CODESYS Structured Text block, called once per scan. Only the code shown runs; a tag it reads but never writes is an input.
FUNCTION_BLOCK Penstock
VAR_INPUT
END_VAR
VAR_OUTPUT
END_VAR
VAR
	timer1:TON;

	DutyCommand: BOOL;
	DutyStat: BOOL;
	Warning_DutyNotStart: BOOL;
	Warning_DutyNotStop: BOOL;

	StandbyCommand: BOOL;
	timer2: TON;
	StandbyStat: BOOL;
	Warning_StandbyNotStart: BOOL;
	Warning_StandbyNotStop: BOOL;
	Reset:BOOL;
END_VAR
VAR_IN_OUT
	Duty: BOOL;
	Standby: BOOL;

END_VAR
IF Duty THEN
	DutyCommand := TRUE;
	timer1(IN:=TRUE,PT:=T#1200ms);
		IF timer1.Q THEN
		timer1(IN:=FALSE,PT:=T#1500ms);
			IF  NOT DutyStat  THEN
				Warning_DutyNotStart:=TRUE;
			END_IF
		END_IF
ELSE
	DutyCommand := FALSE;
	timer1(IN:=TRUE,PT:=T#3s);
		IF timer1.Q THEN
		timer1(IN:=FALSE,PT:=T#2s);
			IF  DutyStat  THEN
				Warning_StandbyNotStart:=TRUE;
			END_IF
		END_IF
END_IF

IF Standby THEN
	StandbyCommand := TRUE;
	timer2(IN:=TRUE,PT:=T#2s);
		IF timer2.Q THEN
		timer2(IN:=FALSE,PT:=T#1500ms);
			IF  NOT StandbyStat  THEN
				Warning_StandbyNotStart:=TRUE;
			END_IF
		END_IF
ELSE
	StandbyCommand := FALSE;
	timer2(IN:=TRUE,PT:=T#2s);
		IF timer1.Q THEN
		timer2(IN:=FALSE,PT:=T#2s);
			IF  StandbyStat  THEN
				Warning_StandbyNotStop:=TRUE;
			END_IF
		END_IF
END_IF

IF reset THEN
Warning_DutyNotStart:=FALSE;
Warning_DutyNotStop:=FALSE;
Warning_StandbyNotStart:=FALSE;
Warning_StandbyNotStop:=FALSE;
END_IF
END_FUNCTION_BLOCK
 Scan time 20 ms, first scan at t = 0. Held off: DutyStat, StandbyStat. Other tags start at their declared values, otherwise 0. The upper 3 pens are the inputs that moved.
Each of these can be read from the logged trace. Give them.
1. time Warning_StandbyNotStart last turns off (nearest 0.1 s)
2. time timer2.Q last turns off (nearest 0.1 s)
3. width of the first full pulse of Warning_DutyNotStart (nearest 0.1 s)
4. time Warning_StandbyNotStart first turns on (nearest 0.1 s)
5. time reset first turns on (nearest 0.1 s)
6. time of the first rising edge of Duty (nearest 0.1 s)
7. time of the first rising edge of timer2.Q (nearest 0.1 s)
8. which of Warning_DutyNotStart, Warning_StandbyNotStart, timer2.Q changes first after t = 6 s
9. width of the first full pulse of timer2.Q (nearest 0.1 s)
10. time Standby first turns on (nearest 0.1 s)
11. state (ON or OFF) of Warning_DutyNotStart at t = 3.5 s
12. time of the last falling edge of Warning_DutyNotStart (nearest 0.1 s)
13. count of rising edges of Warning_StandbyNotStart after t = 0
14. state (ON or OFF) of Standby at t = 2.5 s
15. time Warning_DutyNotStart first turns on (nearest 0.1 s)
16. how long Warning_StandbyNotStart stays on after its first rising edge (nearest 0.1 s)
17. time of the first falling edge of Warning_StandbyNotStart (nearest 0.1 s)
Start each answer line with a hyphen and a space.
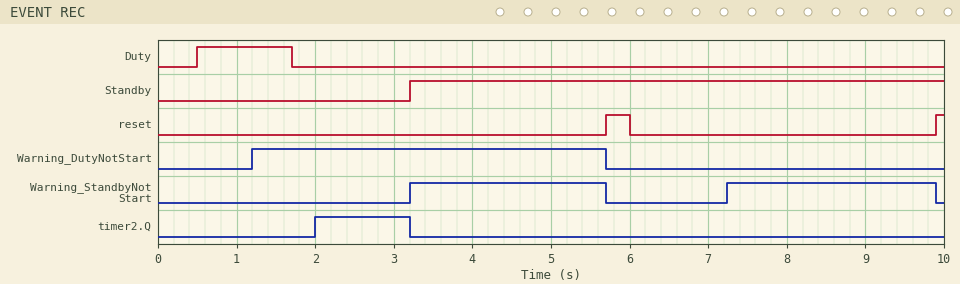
- 9.9 s
- 3.2 s
- 4.5 s
- 3.2 s
- 5.7 s
- 0.5 s
- 2.0 s
- Warning_StandbyNotStart
- 1.2 s
- 3.2 s
- ON
- 5.7 s
- 2
- OFF
- 1.2 s
- 2.5 s
- 5.7 s
